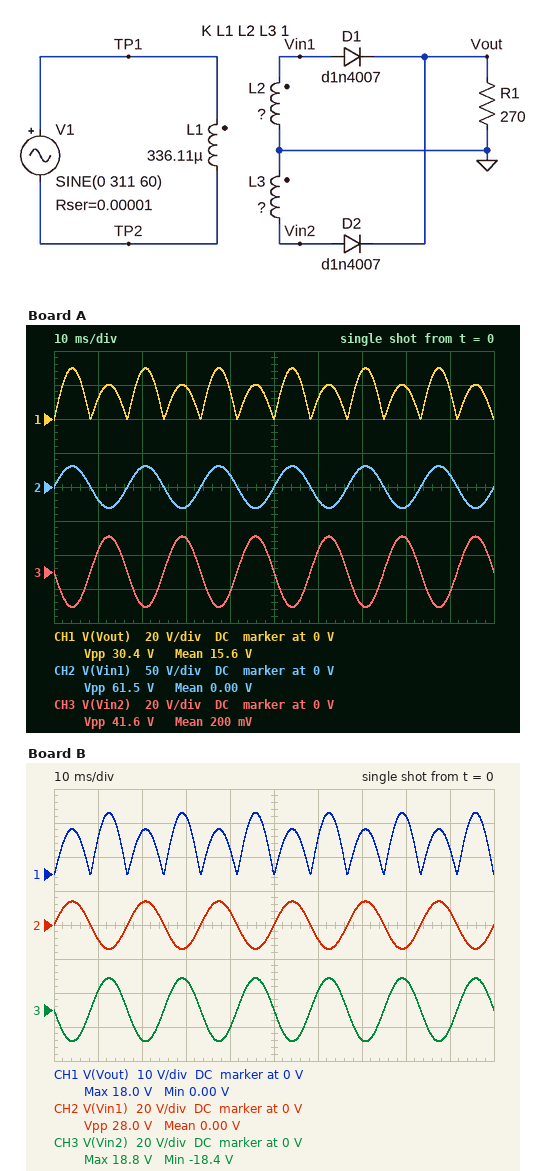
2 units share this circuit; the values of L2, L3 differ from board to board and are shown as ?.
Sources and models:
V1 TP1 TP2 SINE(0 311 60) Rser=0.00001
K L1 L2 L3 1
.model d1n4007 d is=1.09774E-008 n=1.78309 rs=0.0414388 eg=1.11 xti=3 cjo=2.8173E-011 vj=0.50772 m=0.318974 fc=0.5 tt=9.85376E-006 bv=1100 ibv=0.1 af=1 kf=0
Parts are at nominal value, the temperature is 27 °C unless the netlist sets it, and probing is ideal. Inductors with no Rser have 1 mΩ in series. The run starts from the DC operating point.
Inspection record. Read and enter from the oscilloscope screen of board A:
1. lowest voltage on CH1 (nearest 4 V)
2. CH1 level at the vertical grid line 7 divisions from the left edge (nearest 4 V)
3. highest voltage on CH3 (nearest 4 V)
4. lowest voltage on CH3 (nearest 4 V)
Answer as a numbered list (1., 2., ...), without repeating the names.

1. 0 V
2. 28 V
3. 20 V
4. -20 V
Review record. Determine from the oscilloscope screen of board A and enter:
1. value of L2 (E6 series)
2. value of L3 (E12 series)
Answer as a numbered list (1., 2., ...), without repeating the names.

1. 3.3 µH
2. 1.5 µH
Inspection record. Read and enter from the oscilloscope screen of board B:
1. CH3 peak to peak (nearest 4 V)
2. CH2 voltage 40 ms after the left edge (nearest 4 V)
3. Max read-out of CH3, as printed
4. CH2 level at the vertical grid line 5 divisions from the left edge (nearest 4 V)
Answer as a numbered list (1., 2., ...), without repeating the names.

1. 36 V
2. 8 V
3. 18.8 V
4. 0 V
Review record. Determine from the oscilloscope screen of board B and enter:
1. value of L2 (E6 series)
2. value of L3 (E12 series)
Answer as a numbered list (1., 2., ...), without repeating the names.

1. 680 nH
2. 1.2 µH
